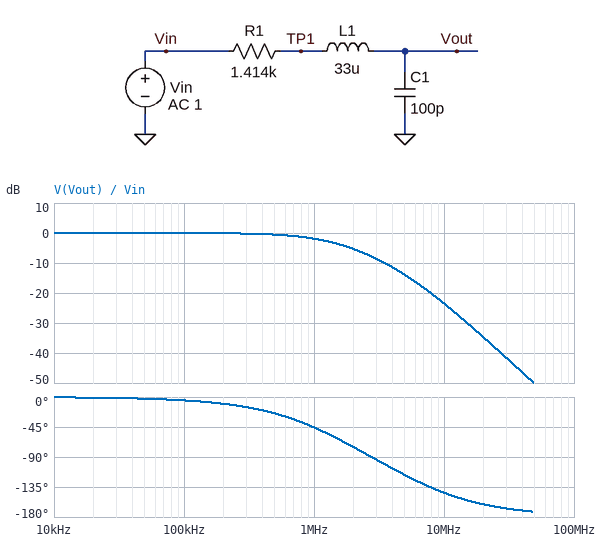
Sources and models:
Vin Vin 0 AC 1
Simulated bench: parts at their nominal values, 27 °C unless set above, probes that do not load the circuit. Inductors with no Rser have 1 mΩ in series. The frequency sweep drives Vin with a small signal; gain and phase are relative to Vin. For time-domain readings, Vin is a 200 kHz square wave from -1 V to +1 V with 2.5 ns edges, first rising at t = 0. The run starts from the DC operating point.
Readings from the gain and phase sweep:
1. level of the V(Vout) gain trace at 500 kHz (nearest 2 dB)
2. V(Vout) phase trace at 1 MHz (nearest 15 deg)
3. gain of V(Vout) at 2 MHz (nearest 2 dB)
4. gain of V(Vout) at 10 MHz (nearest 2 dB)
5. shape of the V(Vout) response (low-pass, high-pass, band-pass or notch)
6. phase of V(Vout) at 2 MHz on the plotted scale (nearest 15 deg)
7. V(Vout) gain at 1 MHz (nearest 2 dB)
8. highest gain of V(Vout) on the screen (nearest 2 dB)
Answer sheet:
0 dB
-45 deg
-6 dB
-24 dB
low-pass
-75 deg
-2 dB
0 dB
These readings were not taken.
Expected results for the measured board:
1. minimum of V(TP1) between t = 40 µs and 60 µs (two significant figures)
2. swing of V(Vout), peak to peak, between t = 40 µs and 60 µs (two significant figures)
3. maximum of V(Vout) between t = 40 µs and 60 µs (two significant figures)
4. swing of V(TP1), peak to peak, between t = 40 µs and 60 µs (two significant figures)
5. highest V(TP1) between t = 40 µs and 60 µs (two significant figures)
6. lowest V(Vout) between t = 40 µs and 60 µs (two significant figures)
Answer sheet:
-1.0 V
2.0 V
1.0 V
2.0 V
1.0 V
-1.0 V
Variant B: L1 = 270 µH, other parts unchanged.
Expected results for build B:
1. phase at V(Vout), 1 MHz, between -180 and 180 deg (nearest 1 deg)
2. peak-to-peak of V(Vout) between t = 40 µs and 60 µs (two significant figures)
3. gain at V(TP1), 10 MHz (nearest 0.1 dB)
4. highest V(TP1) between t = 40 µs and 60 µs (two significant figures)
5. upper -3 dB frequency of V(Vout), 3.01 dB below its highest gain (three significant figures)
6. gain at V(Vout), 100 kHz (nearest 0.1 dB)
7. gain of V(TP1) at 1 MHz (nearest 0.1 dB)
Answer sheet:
-94 deg
2.9 V
0 dB
1.2 V
1.15 MHz
0.1 dB
-22.6 dB
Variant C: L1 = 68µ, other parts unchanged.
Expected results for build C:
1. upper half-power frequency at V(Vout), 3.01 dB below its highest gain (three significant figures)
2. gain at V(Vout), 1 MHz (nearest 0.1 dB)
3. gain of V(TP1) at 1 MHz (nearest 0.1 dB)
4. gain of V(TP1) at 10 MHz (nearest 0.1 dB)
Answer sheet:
1.54 MHz
-1.2 dB
-3.9 dB
-0.5 dB
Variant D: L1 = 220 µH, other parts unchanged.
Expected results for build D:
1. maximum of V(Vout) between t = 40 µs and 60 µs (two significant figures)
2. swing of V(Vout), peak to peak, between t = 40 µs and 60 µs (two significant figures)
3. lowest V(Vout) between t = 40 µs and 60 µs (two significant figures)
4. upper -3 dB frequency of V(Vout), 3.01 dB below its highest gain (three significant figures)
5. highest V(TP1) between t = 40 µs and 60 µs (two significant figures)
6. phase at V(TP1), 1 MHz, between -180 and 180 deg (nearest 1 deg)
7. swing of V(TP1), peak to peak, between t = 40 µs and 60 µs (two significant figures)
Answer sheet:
1.4 V
2.7 V
-1.4 V
1.26 MHz
1.2 V
-82 deg
2.4 V
